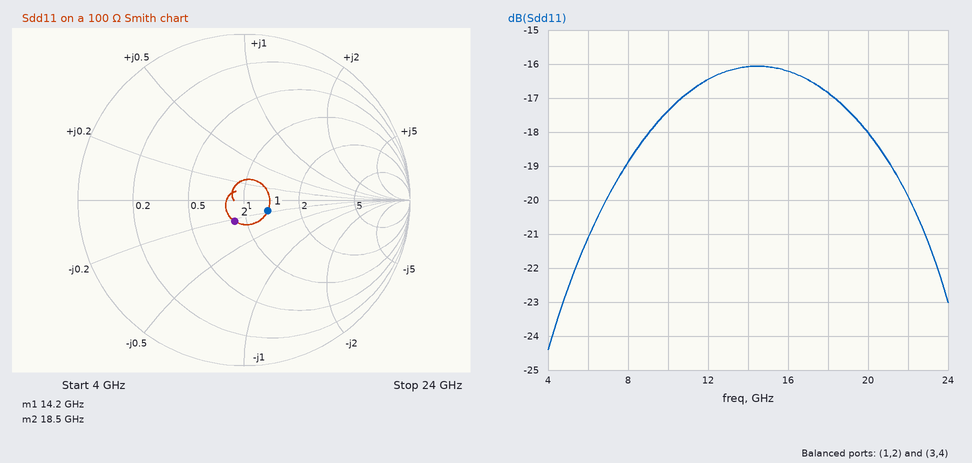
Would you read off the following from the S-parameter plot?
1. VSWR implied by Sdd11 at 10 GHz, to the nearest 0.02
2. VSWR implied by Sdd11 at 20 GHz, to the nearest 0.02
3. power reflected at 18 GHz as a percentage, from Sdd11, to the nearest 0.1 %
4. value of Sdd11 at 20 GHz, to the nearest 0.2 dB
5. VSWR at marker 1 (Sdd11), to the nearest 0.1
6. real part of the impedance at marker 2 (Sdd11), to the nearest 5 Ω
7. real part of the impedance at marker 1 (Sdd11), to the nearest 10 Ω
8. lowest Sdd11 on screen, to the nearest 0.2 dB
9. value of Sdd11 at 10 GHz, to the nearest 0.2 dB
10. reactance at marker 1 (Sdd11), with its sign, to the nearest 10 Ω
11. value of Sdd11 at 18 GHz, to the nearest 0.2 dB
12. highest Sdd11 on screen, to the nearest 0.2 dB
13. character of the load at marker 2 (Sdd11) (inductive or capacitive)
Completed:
1.32
1.28
2.1 %
-18.0 dB
1.4
85 Ω
130 Ω
-24.4 dB
-17.4 dB
-20 Ω
-16.8 dB
-16.0 dB
capacitive
